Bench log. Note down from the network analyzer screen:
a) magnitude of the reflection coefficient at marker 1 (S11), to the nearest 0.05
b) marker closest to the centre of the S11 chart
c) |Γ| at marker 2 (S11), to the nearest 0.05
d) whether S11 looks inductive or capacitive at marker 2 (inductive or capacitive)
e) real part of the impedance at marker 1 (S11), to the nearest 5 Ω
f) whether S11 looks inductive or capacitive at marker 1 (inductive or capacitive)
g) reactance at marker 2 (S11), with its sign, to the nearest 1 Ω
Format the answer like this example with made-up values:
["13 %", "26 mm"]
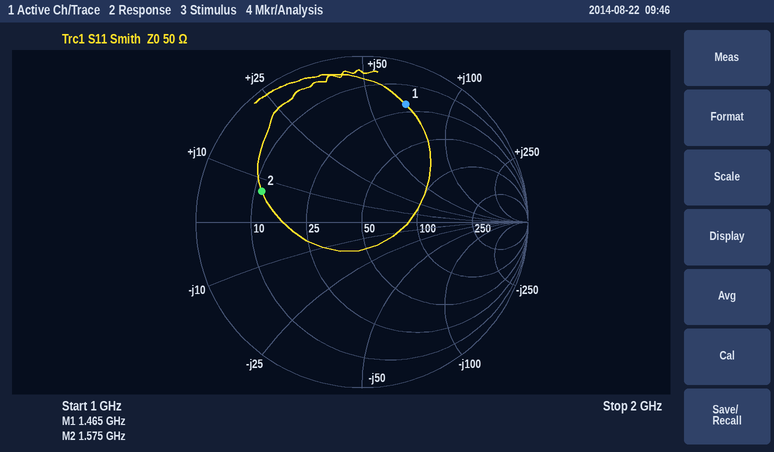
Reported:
["0.75", "marker 2", "0.65", "inductive", "20 Ω", "inductive", "+7 Ω"]
